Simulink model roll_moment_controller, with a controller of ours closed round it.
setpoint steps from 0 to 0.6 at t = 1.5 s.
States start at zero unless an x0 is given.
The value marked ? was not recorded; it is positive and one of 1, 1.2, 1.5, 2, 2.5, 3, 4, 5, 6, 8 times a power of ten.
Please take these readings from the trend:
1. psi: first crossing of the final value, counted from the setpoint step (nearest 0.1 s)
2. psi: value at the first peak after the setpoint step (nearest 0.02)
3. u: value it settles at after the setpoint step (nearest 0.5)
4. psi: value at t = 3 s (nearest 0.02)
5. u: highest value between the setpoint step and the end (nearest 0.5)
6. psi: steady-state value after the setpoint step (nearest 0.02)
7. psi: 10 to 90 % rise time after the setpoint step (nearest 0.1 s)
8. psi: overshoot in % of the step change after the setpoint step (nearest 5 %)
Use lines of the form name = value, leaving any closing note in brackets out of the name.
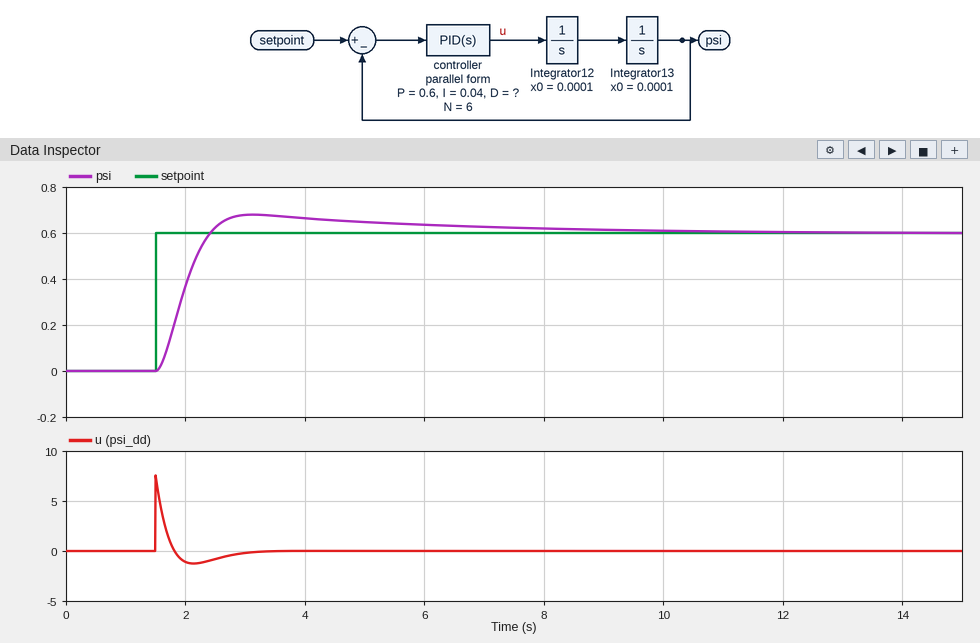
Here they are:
psi: first crossing of the final value, counted from the setpoint step = 0.9 s
psi: value at the first peak after the setpoint step = 0.68
u: value it settles at after the setpoint step = 0.0
psi: value at t = 3 s = 0.68
u: highest value between the setpoint step and the end = 7.5
psi: steady-state value after the setpoint step = 0.60
psi: 10 to 90 % rise time after the setpoint step = 0.6 s
psi: overshoot in % of the step change after the setpoint step = 15 %
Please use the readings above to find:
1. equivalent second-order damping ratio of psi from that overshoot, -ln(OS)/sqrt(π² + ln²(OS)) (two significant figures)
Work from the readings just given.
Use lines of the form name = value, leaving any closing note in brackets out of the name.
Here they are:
equivalent second-order damping ratio of psi from that overshoot, -ln(OS)/sqrt(π² + ln²(OS)) = 0.52
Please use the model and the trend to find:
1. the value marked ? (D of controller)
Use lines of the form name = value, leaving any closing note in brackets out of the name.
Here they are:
the value marked ? = 2
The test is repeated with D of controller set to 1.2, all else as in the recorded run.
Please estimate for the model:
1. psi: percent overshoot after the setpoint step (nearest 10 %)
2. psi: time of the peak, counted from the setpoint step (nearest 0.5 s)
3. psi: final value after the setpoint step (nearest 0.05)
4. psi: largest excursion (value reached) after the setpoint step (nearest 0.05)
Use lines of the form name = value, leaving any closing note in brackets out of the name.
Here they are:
psi: percent overshoot after the setpoint step = 20 %
psi: time of the peak, counted from the setpoint step = 2.5 s
psi: final value after the setpoint step = 0.60
psi: largest excursion (value reached) after the setpoint step = 0.75
